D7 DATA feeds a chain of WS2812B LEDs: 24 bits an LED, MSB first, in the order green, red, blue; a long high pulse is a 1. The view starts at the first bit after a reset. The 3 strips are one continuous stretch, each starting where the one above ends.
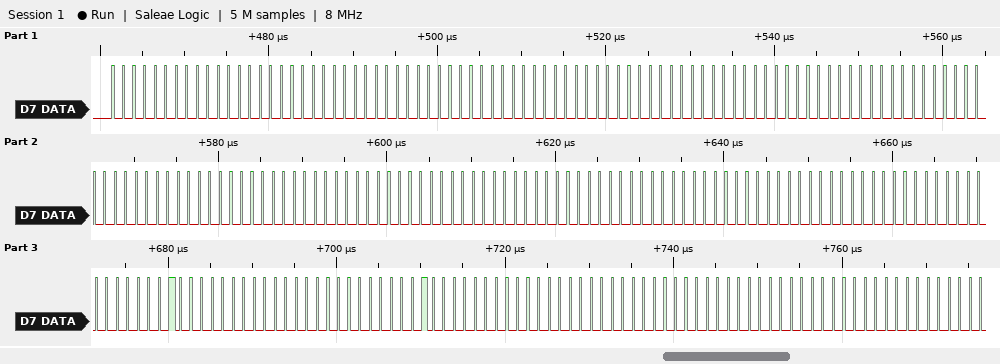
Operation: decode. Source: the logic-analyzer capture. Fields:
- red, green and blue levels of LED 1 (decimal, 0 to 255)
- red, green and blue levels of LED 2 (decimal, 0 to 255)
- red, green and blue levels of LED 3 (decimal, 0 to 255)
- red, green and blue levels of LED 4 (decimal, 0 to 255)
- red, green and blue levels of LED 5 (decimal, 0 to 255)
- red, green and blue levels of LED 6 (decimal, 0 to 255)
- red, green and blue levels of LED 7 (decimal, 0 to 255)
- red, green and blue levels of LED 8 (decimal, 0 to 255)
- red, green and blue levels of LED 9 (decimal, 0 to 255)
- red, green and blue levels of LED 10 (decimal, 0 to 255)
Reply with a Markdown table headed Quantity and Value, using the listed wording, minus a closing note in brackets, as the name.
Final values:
| Quantity | Value |
|---|---|
| red, green and blue levels of LED 1 | 0, 0, 0 |
| red, green and blue levels of LED 2 | 0, 0, 0 |
| red, green and blue levels of LED 3 | 0, 0, 0 |
| red, green and blue levels of LED 4 | 0, 0, 0 |
| red, green and blue levels of LED 5 | 0, 0, 0 |
| red, green and blue levels of LED 6 | 0, 0, 0 |
| red, green and blue levels of LED 7 | 0, 0, 0 |
| red, green and blue levels of LED 8 | 0, 1, 0 |
| red, green and blue levels of LED 9 | 0, 1, 0 |
| red, green and blue levels of LED 10 | 0, 0, 0 |
